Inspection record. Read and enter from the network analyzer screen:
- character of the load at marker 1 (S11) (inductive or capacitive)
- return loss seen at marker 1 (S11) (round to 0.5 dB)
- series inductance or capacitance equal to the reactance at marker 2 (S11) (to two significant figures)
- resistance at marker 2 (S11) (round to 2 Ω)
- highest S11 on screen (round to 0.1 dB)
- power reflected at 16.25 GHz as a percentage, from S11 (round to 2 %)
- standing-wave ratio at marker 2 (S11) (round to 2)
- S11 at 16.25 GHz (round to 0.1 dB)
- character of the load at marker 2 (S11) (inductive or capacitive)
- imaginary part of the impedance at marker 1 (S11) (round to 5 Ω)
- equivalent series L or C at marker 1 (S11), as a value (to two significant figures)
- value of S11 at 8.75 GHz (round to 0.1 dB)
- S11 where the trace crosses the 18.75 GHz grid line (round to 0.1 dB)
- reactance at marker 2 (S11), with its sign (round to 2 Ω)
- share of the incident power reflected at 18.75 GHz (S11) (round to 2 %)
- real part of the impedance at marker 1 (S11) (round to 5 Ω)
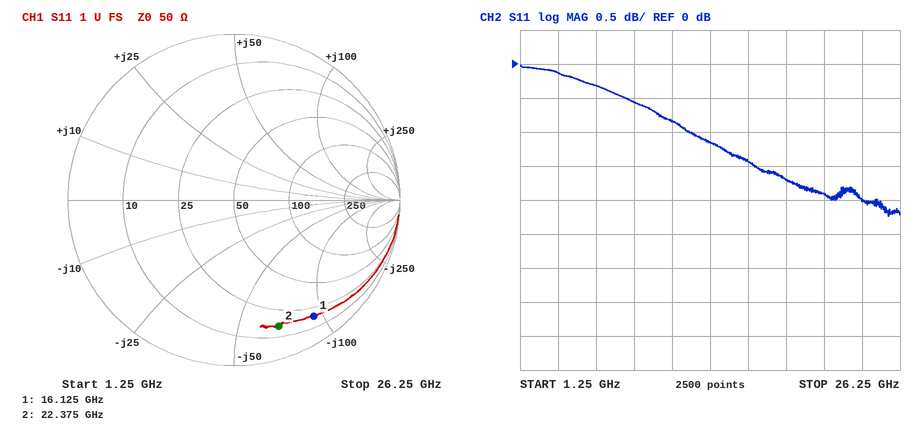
capacitive
1.5 dB
100 fF
16 Ω
0.0 dB
72 %
10
-1.4 dB
capacitive
-90 Ω
110 fF
-0.6 dB
-1.7 dB
-68 Ω
68 %
20 Ω
